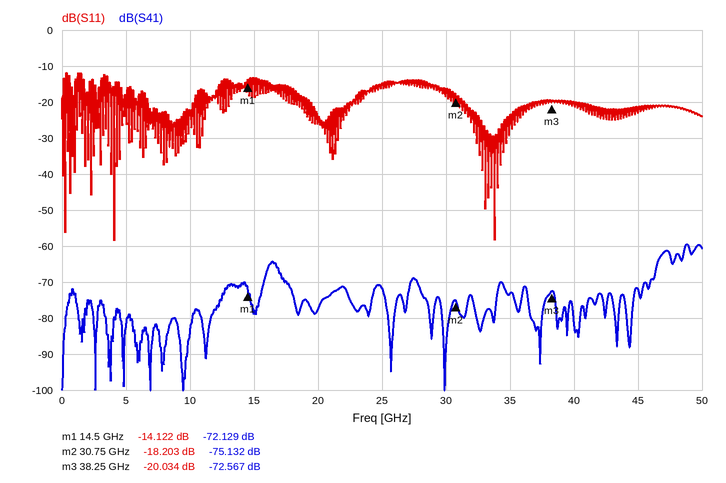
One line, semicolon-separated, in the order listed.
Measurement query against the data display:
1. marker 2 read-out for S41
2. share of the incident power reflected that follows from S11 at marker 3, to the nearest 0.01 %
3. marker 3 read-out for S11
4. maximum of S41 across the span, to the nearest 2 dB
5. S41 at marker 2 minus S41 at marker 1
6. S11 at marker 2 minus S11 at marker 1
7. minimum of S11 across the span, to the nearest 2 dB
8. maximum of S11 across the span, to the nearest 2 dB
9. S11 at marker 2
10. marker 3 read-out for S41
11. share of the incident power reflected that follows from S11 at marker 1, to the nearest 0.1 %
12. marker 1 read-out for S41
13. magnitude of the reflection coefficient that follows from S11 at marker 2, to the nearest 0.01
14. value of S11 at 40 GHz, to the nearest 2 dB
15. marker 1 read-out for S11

-75.132 dB; 0.99 %; -20.034 dB; -60 dB; -3.003 dB; -4.081 dB; -58 dB; -12 dB; -18.203 dB; -72.567 dB; 3.9 %; -72.129 dB; 0.12; -20 dB; -14.122 dB
